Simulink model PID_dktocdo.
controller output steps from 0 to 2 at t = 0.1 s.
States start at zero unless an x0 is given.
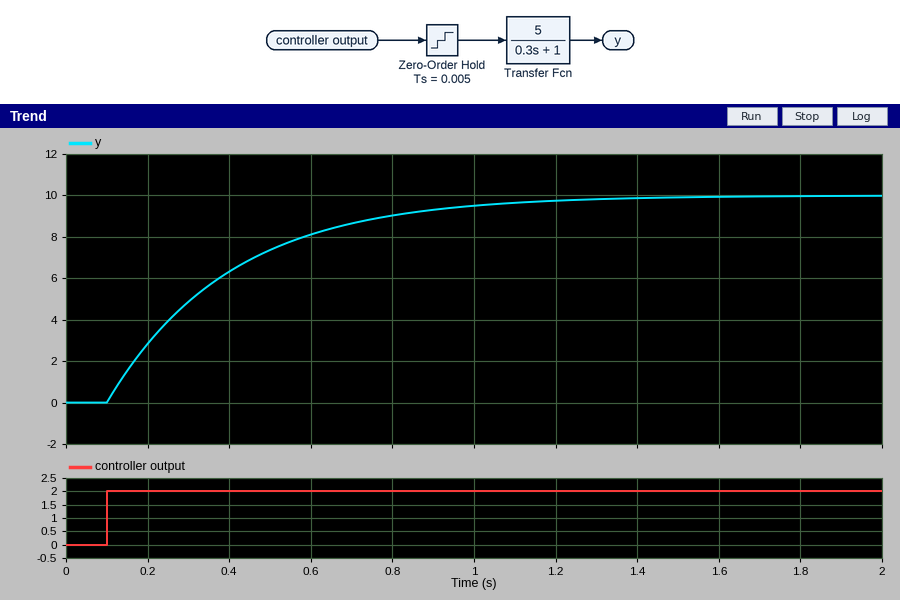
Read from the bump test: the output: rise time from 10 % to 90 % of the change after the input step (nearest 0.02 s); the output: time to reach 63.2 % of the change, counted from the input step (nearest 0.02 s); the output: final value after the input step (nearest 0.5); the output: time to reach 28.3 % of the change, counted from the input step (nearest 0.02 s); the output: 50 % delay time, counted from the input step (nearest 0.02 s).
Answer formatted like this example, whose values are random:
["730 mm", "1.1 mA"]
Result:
["0.66 s", "0.30 s", "10.0", "0.10 s", "0.20 s"]
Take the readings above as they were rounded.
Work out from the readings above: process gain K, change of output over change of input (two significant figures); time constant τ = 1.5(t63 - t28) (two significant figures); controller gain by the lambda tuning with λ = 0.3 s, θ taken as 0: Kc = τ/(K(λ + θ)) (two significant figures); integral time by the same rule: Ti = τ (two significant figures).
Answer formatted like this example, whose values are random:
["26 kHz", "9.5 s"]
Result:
["5.0", "0.30 s", "0.20", "0.30 s"]
